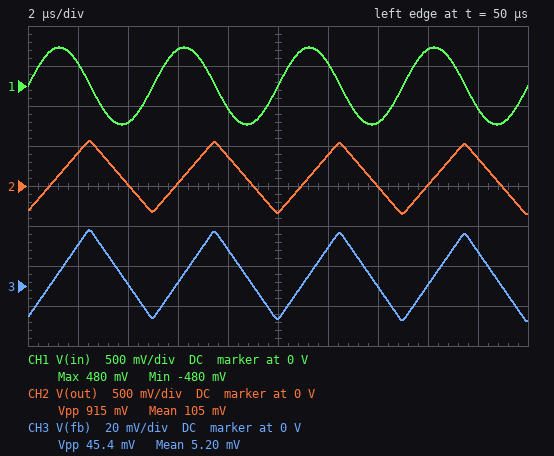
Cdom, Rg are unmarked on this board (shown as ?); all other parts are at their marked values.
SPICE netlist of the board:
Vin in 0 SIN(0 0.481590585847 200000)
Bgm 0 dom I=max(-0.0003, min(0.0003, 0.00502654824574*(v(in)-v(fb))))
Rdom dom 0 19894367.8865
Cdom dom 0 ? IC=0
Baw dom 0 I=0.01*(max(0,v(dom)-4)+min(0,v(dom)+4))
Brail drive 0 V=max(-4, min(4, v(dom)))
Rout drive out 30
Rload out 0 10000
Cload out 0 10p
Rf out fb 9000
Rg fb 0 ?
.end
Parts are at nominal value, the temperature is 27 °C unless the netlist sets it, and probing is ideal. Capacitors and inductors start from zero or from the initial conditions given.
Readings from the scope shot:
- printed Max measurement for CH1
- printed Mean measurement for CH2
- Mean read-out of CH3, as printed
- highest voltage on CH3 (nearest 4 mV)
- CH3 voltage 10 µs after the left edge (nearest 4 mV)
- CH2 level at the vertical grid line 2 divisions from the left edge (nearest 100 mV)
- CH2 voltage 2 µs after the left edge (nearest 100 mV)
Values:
480 mV
105 mV
5.20 mV
28 mV
-16 mV
0 V
400 mV
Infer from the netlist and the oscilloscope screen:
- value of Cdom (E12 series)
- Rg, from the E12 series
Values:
820 pF
470 Ω
